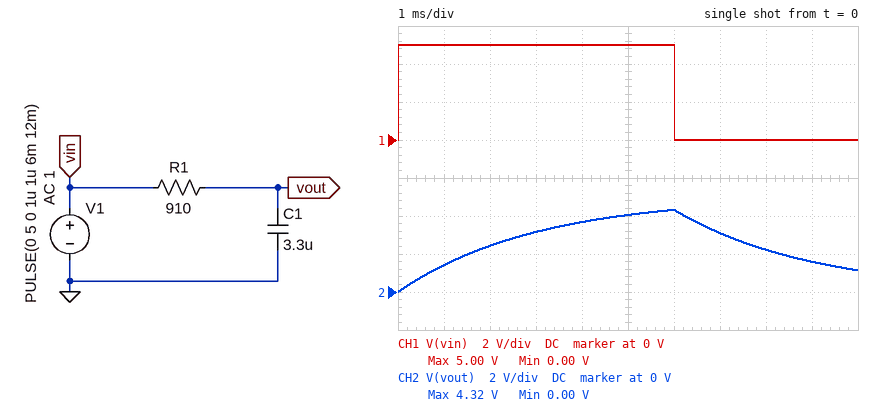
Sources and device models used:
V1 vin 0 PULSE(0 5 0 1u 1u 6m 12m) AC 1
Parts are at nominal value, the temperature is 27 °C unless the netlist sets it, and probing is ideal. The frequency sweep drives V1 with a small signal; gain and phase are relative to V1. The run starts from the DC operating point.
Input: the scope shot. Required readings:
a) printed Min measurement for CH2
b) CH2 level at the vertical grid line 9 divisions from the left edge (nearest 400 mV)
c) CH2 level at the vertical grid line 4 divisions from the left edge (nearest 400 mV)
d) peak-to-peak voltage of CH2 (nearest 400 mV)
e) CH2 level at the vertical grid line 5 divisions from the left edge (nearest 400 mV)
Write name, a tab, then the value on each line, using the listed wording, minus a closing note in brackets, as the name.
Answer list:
printed Min measurement for CH2	0.00 V
CH2 level at the vertical grid line 9 divisions from the left edge	1.6 V
CH2 level at the vertical grid line 4 divisions from the left edge	3.6 V
peak-to-peak voltage of CH2	4.4 V
CH2 level at the vertical grid line 5 divisions from the left edge	4.0 V
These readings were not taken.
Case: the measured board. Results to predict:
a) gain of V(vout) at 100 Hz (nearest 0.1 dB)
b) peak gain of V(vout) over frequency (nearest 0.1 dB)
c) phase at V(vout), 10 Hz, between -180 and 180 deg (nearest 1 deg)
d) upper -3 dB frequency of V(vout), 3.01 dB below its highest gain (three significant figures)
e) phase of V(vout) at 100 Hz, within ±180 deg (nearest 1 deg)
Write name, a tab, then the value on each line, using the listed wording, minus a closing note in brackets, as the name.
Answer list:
gain of V(vout) at 100 Hz	-6.6 dB
peak gain of V(vout) over frequency	0 dB
phase at V(vout), 10 Hz, between -180 and 180 deg	-11 deg
upper -3 dB frequency of V(vout), 3.01 dB below its highest gain	53.0 Hz
phase of V(vout) at 100 Hz, within ±180 deg	-62 deg
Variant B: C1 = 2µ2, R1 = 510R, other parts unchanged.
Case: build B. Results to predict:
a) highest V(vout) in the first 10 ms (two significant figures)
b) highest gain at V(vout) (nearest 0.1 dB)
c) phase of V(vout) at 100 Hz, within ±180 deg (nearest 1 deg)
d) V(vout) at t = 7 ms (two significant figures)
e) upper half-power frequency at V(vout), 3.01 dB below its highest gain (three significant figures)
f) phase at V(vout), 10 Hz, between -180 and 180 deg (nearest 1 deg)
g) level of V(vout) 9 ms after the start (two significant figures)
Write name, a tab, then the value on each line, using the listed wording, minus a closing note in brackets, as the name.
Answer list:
highest V(vout) in the first 10 ms	5.0 V
highest gain at V(vout)	0 dB
phase of V(vout) at 100 Hz, within ±180 deg	-35 deg
V(vout) at t = 7 ms	2.0 V
upper half-power frequency at V(vout), 3.01 dB below its highest gain	142 Hz
phase at V(vout), 10 Hz, between -180 and 180 deg	-4 deg
level of V(vout) 9 ms after the start	340 mV
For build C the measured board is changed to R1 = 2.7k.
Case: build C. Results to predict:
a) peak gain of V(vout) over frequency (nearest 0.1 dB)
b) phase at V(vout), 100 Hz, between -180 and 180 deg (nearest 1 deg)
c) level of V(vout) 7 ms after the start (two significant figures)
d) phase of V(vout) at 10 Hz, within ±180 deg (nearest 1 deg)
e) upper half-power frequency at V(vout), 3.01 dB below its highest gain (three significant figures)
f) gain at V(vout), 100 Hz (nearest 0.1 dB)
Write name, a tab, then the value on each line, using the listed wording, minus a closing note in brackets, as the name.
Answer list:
peak gain of V(vout) over frequency	0 dB
phase at V(vout), 100 Hz, between -180 and 180 deg	-80 deg
level of V(vout) 7 ms after the start	2.2 V
phase of V(vout) at 10 Hz, within ±180 deg	-29 deg
upper half-power frequency at V(vout), 3.01 dB below its highest gain	17.9 Hz
gain at V(vout), 100 Hz	-15.1 dB
